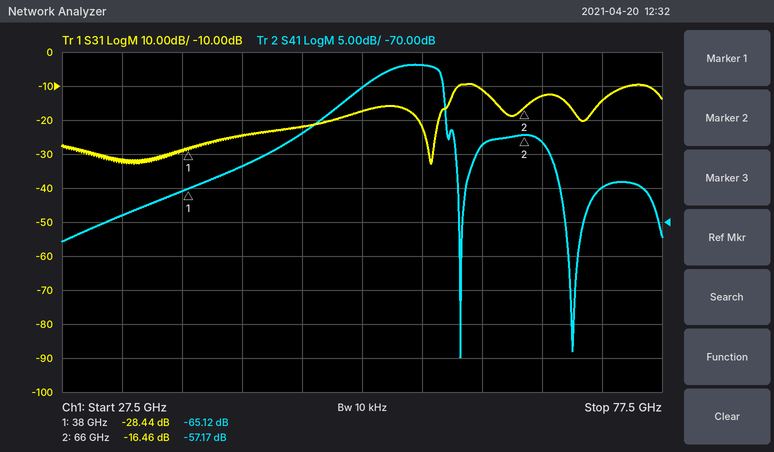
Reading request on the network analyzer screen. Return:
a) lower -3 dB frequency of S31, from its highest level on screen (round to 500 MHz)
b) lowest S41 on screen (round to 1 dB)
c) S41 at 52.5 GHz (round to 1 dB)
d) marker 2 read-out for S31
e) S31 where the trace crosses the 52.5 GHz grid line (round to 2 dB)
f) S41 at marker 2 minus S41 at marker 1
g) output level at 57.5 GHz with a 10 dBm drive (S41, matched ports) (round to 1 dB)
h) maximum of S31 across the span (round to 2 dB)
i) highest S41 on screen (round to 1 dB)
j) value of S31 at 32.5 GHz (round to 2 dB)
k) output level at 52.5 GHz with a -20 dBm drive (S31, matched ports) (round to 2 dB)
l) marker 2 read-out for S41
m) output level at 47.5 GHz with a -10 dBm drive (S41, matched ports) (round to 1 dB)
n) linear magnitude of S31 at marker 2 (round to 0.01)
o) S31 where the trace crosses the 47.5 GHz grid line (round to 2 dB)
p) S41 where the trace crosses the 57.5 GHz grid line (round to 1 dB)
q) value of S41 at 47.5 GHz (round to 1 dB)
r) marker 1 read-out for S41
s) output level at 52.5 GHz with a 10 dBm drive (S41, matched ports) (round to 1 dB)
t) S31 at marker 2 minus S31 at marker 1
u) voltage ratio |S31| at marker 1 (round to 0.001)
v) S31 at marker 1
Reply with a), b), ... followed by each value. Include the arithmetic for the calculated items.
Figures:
a) 60.0 GHz
b) -90 dB
c) -50 dB
d) -16.46 dB
e) -18 dB
f) -57.17 − (-65.12) = 7.95 dB
g) 10 dBm + (-47 dB) = -37 dBm
h) -10 dB
i) -47 dB
j) -32 dB
k) -20 dBm + (-18 dB) = -38 dBm
l) -57.17 dB
m) -10 dBm + (-57 dB) = -67 dBm
n) 10^(-16.46/20) ≈ 0.15
o) -22 dB
p) -47 dB
q) -57 dB
r) -65.12 dB
s) 10 dBm + (-50 dB) = -40 dBm
t) -16.46 − (-28.44) = 11.98 dB
u) 10^(-28.44/20) ≈ 0.038
v) -28.44 dB
